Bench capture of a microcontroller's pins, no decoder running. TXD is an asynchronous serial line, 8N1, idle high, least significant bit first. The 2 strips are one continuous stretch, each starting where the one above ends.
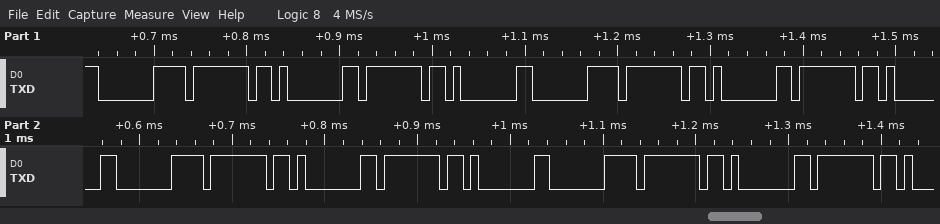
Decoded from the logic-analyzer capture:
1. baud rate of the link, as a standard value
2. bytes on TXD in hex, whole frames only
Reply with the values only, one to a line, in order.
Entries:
115200 baud
C0 7F 01 7F 01 C0 7F 01 7F 01 C0 7F 01 7F 01 C0 7F 01 7F
